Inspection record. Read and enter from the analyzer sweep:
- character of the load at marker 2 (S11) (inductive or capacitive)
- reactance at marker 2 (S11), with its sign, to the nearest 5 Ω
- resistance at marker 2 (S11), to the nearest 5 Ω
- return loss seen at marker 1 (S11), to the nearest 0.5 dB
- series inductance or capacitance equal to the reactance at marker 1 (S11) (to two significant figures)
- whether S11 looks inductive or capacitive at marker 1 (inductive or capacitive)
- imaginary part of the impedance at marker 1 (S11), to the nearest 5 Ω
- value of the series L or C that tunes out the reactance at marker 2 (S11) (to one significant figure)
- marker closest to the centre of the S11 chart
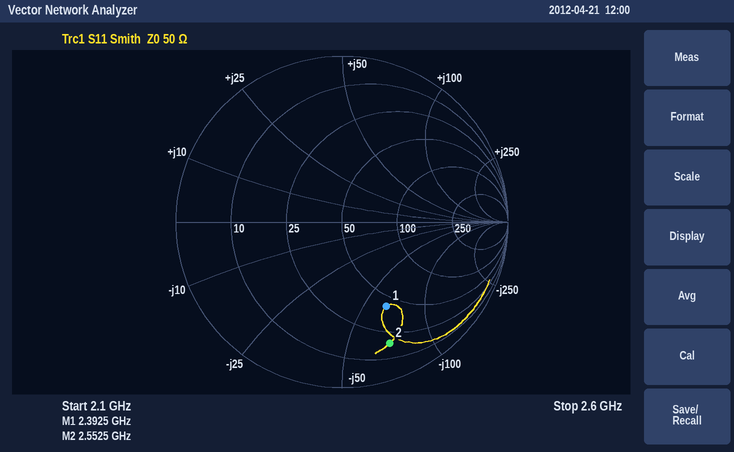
capacitive
-70 Ω
20 Ω
5.0 dB
1.0 pF
capacitive
-65 Ω
4 nH
marker 1
